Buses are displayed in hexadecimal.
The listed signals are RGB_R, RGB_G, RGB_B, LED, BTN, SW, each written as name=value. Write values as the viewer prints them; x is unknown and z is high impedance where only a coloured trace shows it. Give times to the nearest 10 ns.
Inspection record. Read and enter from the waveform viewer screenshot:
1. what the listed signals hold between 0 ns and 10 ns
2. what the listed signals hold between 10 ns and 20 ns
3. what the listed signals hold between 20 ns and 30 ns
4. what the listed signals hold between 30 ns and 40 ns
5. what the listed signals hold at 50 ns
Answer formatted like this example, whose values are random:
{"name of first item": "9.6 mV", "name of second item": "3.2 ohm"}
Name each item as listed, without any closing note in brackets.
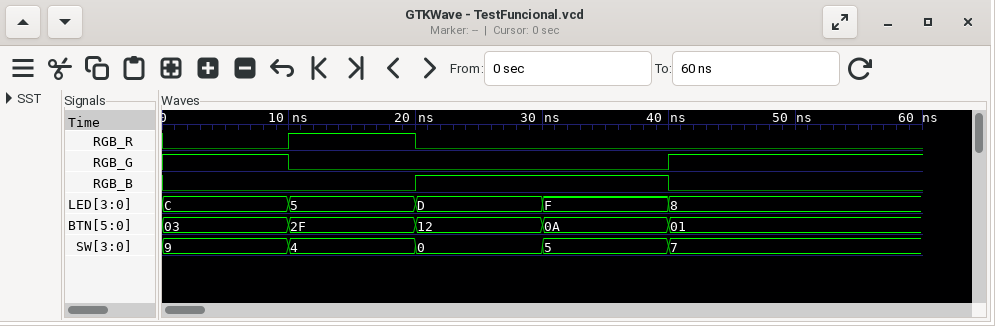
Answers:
{"what the listed signals hold between 0 ns and 10 ns": "RGB_R=0, RGB_G=1, RGB_B=0, LED=C, BTN=03, SW=9", "what the listed signals hold between 10 ns and 20 ns": "RGB_R=1, RGB_G=0, RGB_B=0, LED=5, BTN=2F, SW=4", "what the listed signals hold between 20 ns and 30 ns": "RGB_R=0, RGB_G=0, RGB_B=1, LED=D, BTN=12, SW=0", "what the listed signals hold between 30 ns and 40 ns": "RGB_R=0, RGB_G=0, RGB_B=1, LED=F, BTN=0A, SW=5", "what the listed signals hold at 50 ns": "RGB_R=0, RGB_G=1, RGB_B=0, LED=8, BTN=01, SW=7"}
